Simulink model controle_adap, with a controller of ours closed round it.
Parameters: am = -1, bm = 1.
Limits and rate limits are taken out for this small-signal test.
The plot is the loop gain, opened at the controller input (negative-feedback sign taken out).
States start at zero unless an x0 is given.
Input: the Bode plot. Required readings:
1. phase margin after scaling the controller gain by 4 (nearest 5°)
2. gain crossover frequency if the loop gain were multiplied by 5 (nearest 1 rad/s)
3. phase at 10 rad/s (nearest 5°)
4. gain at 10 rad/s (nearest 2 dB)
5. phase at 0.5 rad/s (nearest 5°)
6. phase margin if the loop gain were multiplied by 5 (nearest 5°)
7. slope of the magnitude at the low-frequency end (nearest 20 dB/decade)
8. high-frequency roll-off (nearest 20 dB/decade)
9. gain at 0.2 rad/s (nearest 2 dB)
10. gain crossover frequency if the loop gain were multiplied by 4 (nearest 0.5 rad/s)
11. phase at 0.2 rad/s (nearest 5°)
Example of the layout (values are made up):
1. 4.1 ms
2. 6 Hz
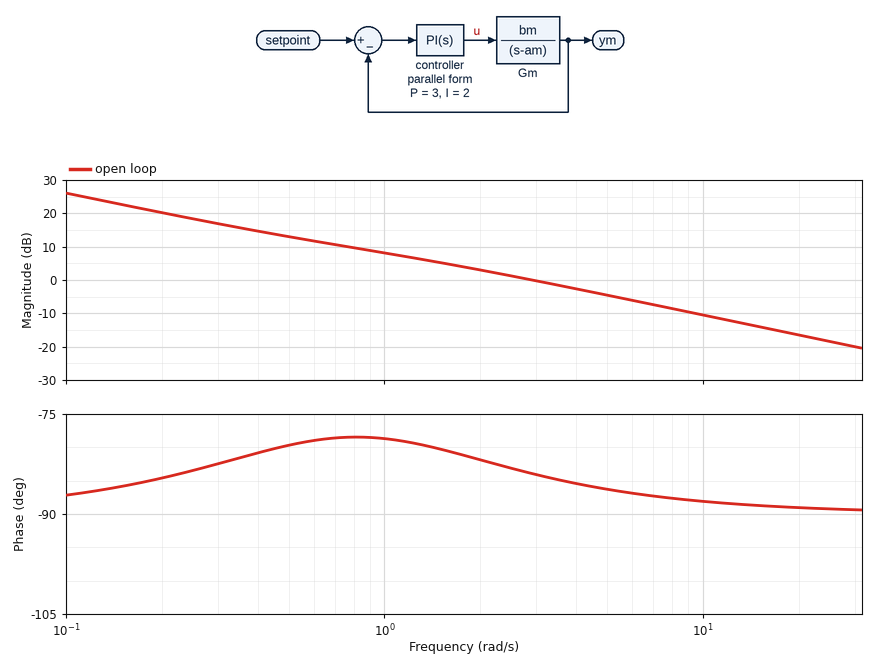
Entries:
1. 90°
2. 15 rad/s
3. -90°
4. -10 dB
5. -80°
6. 90°
7. -20 dB/decade
8. -20 dB/decade
9. 20 dB
10. 12.0 rad/s
11. -85°
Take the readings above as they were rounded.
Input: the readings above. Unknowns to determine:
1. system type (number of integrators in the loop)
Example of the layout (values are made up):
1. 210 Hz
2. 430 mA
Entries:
1. 1
